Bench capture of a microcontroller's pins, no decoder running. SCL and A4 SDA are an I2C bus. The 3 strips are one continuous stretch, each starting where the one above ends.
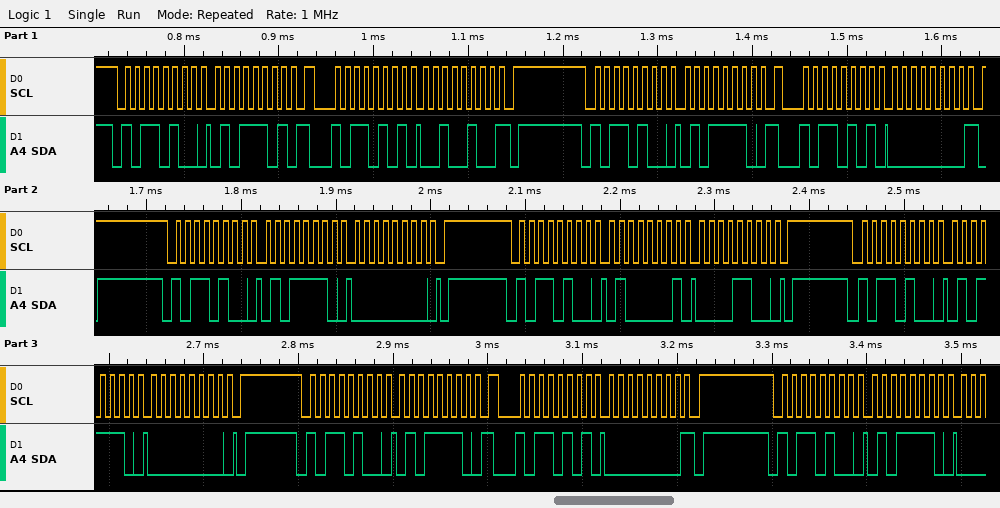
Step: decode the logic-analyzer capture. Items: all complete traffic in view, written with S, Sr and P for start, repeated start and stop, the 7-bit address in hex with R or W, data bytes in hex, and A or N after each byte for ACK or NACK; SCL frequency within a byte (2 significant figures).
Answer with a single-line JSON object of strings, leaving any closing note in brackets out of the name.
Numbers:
{"all complete traffic in view, written with S, Sr and P for start, repeated start and stop, the 7-bit address in hex with R or W, data bytes in hex, and A or N after each byte for ACK or NACK": "S 5AW A 5D A Sr 5AR A 24 N P S 5AW A 5E A Sr 5AR A 00 N P S 5AW A 5E A 00 A P S 5AW A 41 A 0C A P S 5AW A 5E A 00 A P S 5AW A 5E A Sr 5AR A 00 N P S 5AW A 5E A", "SCL frequency within a byte": "100 kHz"}
